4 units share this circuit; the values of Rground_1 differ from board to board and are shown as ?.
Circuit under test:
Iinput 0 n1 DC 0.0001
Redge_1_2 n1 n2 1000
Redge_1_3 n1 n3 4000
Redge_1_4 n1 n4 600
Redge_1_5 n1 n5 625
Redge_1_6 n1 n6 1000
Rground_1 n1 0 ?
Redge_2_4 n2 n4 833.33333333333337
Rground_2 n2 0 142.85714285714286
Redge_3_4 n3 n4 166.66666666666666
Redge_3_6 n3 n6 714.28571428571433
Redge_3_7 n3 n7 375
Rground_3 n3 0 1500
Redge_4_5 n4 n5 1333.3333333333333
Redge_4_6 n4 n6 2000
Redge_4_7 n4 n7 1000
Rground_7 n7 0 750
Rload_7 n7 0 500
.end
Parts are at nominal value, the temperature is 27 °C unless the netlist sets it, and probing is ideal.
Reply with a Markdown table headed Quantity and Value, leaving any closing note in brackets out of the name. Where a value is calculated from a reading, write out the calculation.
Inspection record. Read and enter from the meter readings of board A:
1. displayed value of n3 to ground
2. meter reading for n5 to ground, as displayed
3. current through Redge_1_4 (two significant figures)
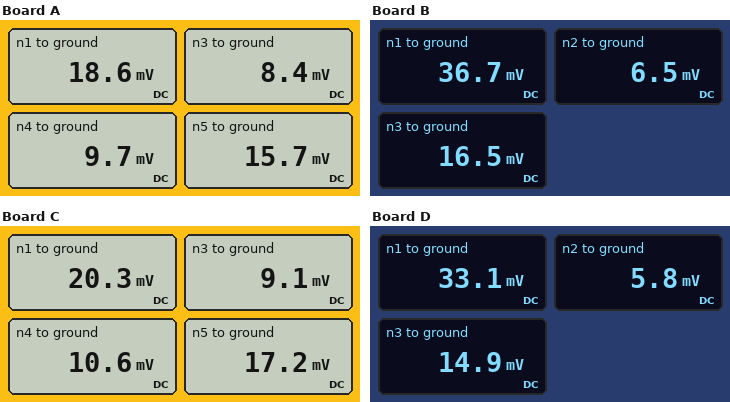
| Quantity | Value |
|---|---|
| displayed value of n3 to ground | 8.4 mV |
| meter reading for n5 to ground, as displayed | 15.7 mV |
| current through Redge_1_4 | (18.6 mV - 9.7 mV) / 600 Ω = 15 µA |
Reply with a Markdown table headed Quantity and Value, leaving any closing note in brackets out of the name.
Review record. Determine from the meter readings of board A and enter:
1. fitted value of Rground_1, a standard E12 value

| Quantity | Value |
|---|---|
| fitted value of Rground_1, a standard E12 value | 330 Ω |
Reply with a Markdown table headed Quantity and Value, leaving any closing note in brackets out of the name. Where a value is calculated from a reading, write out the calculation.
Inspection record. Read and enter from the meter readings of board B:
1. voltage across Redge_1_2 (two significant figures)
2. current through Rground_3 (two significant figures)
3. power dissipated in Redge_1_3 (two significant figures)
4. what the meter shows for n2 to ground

| Quantity | Value |
|---|---|
| voltage across Redge_1_2 | 36.7 mV - 6.5 mV = 30 mV |
| current through Rground_3 | (16.5 mV) / 1.5 kΩ = 11 µA |
| power dissipated in Redge_1_3 | (36.7 mV - 16.5 mV)^2 / 4 kΩ = 100 nW |
| what the meter shows for n2 to ground | 6.5 mV |
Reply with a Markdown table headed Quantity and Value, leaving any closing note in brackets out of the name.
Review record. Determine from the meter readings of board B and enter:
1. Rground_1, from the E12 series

| Quantity | Value |
|---|---|
| Rground_1, from the E12 series | 2.7 kΩ |
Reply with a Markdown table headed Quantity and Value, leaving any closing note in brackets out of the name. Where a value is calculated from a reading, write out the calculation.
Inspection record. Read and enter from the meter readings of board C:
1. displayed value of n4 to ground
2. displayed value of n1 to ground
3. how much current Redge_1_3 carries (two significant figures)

| Quantity | Value |
|---|---|
| displayed value of n4 to ground | 10.6 mV |
| displayed value of n1 to ground | 20.3 mV |
| how much current Redge_1_3 carries | (20.3 mV - 9.1 mV) / 4 kΩ = 2.8 µA |
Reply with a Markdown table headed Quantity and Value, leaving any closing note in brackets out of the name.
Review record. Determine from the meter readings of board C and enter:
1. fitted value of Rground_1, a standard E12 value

| Quantity | Value |
|---|---|
| fitted value of Rground_1, a standard E12 value | 390 Ω |
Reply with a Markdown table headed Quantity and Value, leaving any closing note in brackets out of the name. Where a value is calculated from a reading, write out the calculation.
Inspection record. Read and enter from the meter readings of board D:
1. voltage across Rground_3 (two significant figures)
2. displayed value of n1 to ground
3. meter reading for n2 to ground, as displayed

| Quantity | Value |
|---|---|
| voltage across Rground_3 | 14.9 mV = 15 mV |
| displayed value of n1 to ground | 33.1 mV |
| meter reading for n2 to ground, as displayed | 5.8 mV |
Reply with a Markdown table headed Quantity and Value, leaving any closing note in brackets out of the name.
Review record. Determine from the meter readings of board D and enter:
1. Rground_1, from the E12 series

| Quantity | Value |
|---|---|
| Rground_1, from the E12 series | 1.5 kΩ |
